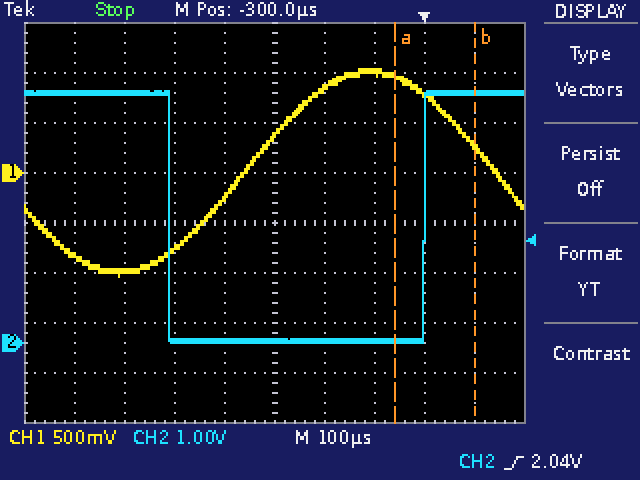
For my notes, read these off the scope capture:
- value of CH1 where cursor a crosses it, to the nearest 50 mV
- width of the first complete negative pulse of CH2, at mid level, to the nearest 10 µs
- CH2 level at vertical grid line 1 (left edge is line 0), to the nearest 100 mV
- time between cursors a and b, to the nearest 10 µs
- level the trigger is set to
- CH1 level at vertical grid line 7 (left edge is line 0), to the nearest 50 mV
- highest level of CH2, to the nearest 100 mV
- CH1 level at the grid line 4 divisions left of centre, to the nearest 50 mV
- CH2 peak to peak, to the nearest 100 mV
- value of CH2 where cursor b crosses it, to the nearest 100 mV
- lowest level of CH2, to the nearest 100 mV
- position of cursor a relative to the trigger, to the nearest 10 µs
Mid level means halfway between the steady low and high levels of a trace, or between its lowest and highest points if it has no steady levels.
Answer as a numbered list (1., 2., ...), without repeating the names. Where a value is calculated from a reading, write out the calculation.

1. 950 mV
2. 510 µs
3. 5.0 V
4. 160 µs
5. 2.04 V
6. 1.00 V
7. 5.0 V
8. -850 mV
9. 5.0 V − (0.0 V) = 5.0 V
10. 5.0 V
11. 0.0 V
12. -60 µs
